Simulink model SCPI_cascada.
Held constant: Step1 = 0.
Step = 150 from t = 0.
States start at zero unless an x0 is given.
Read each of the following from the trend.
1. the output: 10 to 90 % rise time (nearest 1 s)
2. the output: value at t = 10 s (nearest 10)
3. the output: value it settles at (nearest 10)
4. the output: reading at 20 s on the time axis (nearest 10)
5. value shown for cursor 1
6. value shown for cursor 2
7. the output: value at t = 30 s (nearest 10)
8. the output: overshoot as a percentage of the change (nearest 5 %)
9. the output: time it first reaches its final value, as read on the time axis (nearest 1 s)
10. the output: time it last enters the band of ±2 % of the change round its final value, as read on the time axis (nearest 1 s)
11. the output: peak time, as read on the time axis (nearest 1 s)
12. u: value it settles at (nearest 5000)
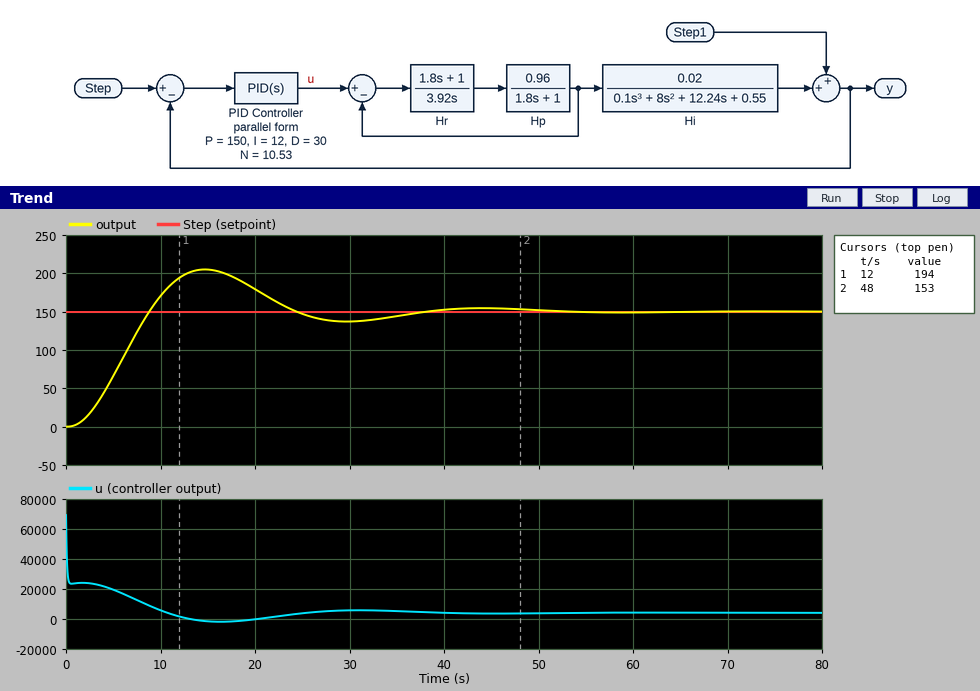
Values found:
6 s
170
150
180
194
153
140
35 %
9 s
48 s
15 s
5000
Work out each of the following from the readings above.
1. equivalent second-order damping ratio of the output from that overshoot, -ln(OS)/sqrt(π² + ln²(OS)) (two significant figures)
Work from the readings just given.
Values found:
0.32
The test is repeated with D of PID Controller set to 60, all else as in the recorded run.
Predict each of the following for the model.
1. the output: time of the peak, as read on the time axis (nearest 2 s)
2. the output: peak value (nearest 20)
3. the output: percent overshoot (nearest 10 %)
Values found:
14 s
200
30 %
